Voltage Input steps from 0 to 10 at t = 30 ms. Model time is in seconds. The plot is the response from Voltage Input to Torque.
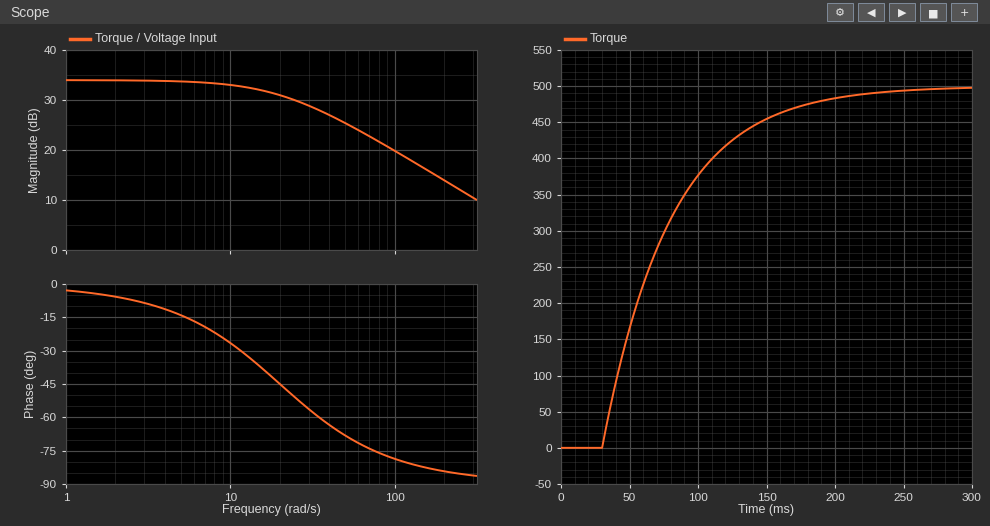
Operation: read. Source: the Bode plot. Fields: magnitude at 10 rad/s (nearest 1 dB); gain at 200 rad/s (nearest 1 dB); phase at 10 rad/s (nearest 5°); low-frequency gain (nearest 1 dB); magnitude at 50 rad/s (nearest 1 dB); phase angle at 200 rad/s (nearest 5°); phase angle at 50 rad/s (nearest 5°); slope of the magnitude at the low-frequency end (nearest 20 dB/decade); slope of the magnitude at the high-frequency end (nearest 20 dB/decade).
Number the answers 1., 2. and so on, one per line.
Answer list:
1. 33 dB
2. 14 dB
3. -25°
4. 34 dB
5. 25 dB
6. -85°
7. -70°
8. 0 dB/decade
9. -20 dB/decade
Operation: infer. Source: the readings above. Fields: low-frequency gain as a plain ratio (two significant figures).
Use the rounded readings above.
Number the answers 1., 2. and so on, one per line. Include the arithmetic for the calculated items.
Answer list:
1. 10^(34 / 20) = 50
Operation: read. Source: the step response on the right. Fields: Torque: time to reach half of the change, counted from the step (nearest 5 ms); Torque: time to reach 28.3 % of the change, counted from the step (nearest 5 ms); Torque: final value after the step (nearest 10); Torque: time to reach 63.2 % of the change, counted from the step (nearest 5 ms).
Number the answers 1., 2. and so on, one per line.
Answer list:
1. 35 ms
2. 15 ms
3. 500
4. 50 ms
